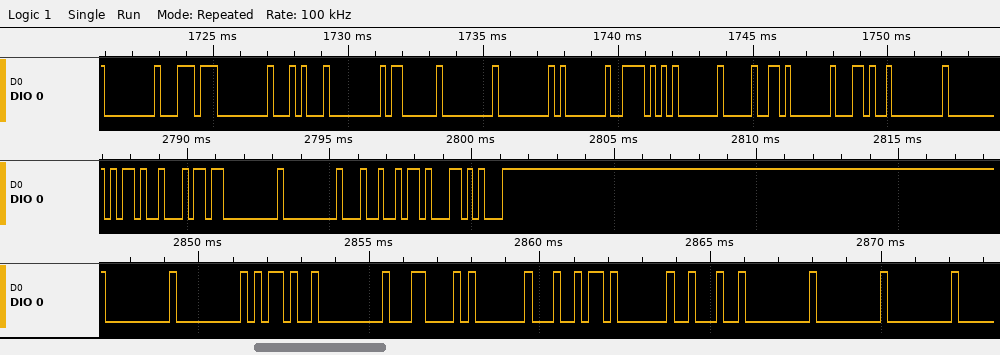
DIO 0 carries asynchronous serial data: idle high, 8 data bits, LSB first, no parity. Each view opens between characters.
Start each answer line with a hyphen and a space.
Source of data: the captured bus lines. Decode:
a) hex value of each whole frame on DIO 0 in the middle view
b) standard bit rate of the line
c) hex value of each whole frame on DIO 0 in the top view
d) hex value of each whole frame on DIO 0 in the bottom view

- 2D, B4, 00, 00, 24, 8B, C5
- 4800 baud
- 00, DC, 00, 14, 00, 03, 00, 00, 01, 5E, 01, 90, 01, 2C, 00
- 00, 00, 2D, 00, 0C, 01, A4, 01, 22, 00, 00, 00
